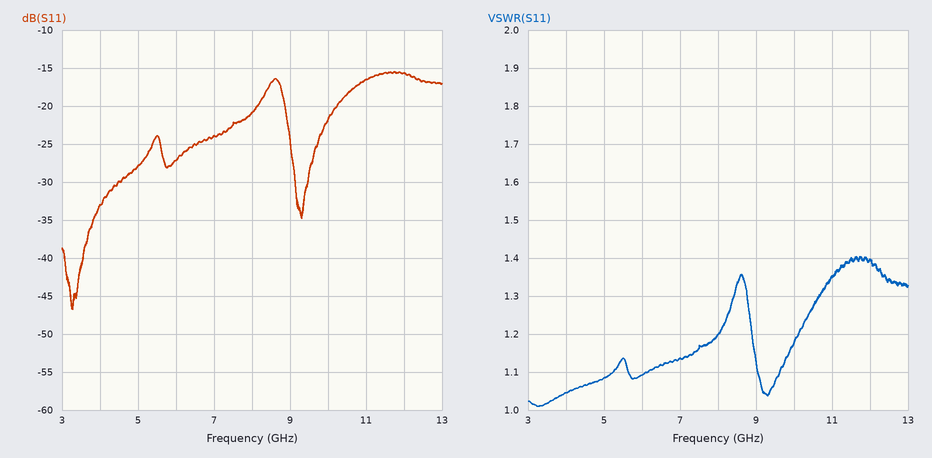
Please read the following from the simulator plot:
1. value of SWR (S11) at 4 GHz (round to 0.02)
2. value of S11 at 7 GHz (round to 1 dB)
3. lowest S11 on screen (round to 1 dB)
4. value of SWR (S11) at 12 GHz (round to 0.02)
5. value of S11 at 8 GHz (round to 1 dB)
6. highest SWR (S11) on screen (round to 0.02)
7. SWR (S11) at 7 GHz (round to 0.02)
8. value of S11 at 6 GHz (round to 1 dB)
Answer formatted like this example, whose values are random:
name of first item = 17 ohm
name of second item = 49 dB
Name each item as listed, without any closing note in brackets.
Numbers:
value of SWR (S11) at 4 GHz = 1.04
value of S11 at 7 GHz = -24 dB
lowest S11 on screen = -47 dB
value of SWR (S11) at 12 GHz = 1.40
value of S11 at 8 GHz = -21 dB
highest SWR (S11) on screen = 1.40
SWR (S11) at 7 GHz = 1.14
value of S11 at 6 GHz = -27 dB
